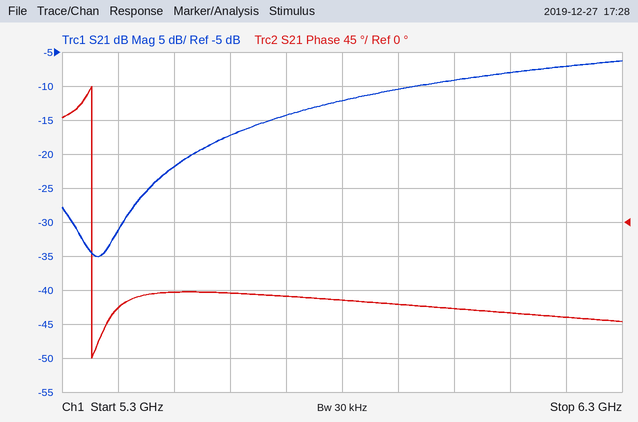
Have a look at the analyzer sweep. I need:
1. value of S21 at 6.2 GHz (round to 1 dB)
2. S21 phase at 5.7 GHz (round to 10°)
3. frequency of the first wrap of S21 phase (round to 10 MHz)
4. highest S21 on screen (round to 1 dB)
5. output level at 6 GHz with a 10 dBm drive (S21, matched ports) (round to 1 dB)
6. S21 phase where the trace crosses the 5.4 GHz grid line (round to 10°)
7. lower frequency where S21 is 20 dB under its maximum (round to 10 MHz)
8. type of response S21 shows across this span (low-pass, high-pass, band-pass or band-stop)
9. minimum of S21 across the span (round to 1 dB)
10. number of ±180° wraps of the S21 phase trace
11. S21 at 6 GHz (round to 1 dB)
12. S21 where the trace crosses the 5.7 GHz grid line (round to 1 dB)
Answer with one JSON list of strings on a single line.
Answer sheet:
["-7 dB", "-100°", "5.35 GHz", "-6 dB", "1 dBm", "-110°", "5.44 GHz", "high-pass", "-35 dB", "1", "-9 dB", "-14 dB"]
